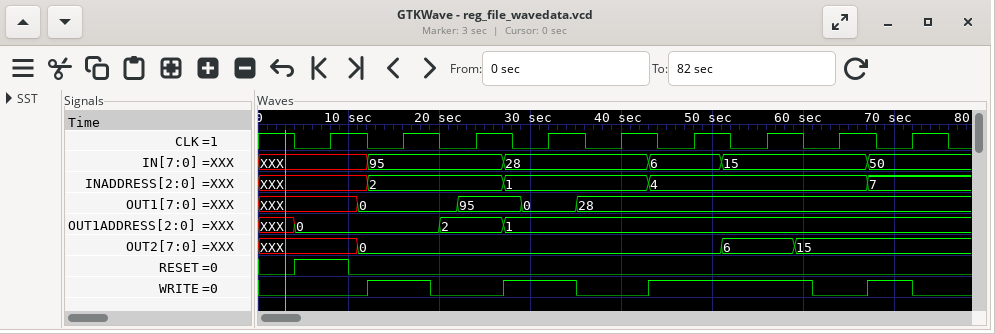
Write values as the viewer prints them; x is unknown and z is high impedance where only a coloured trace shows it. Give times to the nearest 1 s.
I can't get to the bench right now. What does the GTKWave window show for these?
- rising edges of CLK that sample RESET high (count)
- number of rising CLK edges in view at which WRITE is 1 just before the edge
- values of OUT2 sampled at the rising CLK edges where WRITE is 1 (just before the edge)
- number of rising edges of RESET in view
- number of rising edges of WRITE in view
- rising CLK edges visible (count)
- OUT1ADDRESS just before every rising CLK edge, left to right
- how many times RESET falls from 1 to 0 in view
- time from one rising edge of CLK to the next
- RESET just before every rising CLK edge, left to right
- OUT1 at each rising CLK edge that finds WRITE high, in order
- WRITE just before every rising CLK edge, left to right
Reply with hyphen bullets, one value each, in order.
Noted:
- 1
- 5
- 0, 0, 0, 6, 15
- 1
- 4
- 9
- 0, 0, 2, 1, 1, 1, 1, 1, 1
- 1
- 8 s
- 1 0 0 0 0 0 0 0 0
- 0, 0, 28, 28, 28
- 0 1 0 1 0 1 1 0 1
